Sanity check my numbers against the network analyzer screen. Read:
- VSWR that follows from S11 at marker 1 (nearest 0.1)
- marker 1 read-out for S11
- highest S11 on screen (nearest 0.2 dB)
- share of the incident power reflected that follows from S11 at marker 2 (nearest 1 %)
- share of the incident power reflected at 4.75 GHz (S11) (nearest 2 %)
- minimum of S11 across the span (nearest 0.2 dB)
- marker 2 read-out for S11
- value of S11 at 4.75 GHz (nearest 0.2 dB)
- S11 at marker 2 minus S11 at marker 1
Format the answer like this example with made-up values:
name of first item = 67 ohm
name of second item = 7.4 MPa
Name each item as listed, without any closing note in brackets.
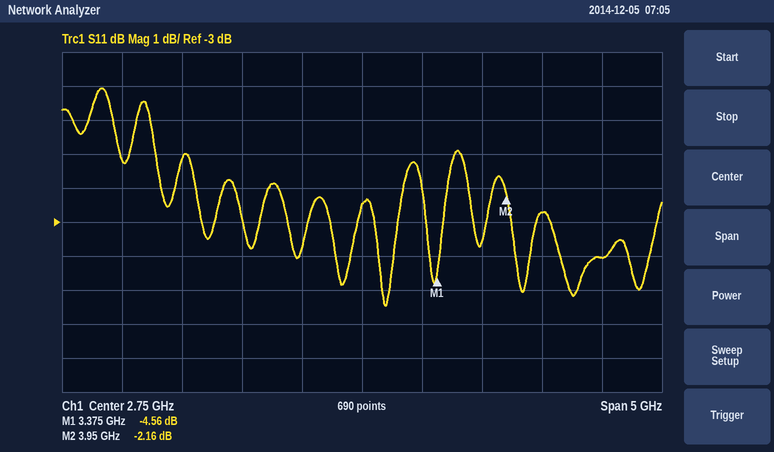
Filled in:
VSWR that follows from S11 at marker 1 = 3.9
marker 1 read-out for S11 = -4.56 dB
highest S11 on screen = 1.0 dB
share of the incident power reflected that follows from S11 at marker 2 = 61 %
share of the incident power reflected at 4.75 GHz (S11) = 40 %
minimum of S11 across the span = -5.4 dB
marker 2 read-out for S11 = -2.16 dB
value of S11 at 4.75 GHz = -4.0 dB
S11 at marker 2 minus S11 at marker 1 = 2.40 dB
